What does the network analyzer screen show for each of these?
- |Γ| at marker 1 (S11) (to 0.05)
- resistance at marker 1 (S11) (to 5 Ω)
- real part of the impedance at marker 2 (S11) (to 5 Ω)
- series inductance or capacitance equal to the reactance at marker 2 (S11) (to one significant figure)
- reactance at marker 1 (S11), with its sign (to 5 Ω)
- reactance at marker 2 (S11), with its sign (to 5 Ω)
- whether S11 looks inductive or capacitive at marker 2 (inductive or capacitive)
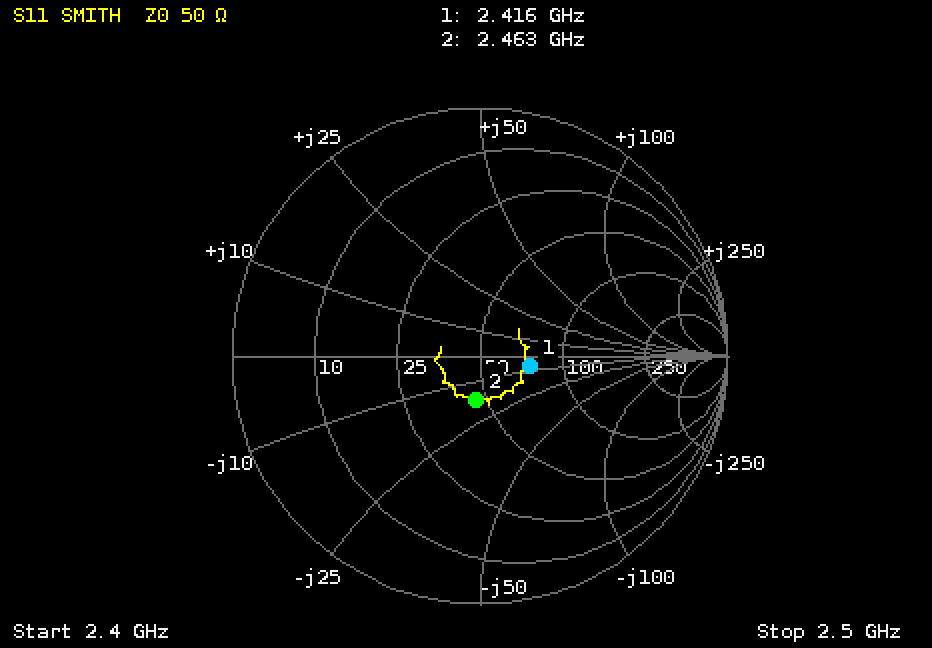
0.20
75 Ω
45 Ω
4 pF
-5 Ω
-15 Ω
capacitive
